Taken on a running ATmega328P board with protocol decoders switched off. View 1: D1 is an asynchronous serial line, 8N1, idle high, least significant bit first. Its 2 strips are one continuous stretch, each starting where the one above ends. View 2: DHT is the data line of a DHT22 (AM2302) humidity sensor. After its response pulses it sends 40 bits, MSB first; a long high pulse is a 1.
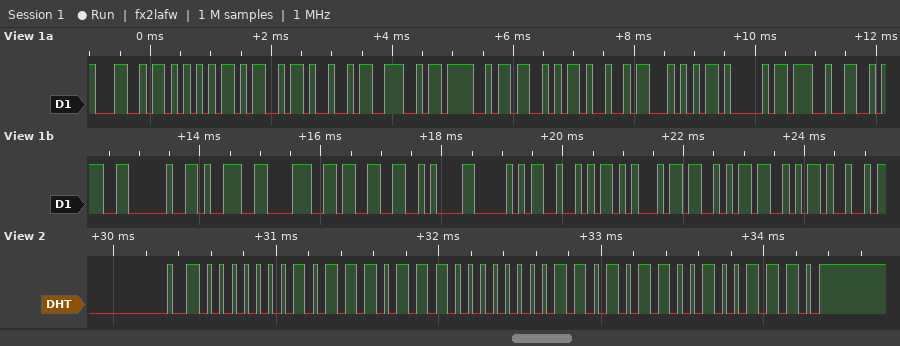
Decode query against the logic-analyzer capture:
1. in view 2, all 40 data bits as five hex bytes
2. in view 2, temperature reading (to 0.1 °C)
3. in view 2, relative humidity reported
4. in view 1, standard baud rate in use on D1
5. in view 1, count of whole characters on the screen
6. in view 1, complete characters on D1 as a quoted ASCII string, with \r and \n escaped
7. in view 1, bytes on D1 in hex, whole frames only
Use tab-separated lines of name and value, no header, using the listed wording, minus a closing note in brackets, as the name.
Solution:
in view 2, all 40 data bits as five hex bytes	01 77 00 D6 4E
in view 2, temperature reading	21.4 °C
in view 2, relative humidity reported	37.5 %
in view 1, standard baud rate in use on D1	9600 baud
in view 1, count of whole characters on the screen	23
in view 1, complete characters on D1 as a quoted ASCII string, with \r and \n escaped	"LUMINOSITA': 983\nPRESSI"
in view 1, bytes on D1 in hex, whole frames only	4C 55 4D 49 4E 4F 53 49 54 41 27 3A 20 39 38 33 0A 50 52 45 53 53 49
